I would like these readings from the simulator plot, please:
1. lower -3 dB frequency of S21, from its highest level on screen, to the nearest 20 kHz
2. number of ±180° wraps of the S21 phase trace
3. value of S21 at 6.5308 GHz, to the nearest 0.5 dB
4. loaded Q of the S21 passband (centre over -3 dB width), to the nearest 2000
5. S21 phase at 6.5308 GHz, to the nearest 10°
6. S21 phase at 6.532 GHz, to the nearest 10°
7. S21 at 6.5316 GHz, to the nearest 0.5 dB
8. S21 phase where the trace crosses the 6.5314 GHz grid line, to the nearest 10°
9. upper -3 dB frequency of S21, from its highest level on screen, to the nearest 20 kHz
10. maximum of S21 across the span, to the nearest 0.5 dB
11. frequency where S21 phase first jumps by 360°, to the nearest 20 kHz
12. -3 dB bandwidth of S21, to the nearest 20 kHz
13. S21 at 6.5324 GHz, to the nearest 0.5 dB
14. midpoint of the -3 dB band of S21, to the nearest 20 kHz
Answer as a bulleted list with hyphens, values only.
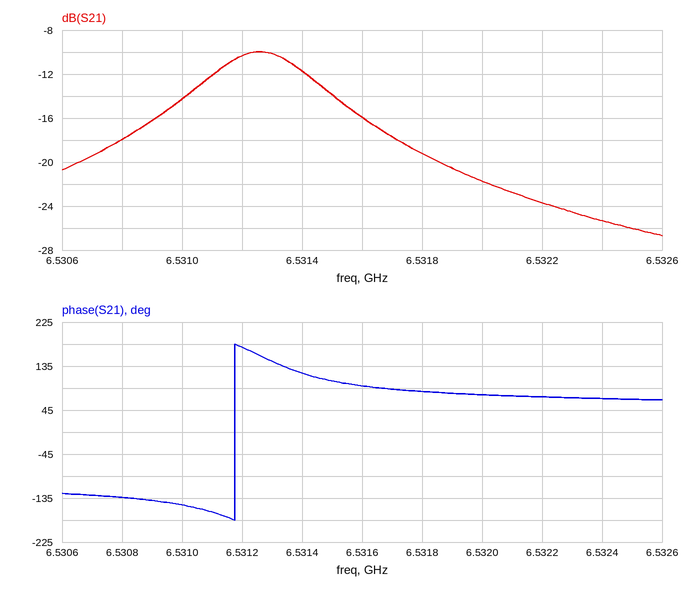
- 6.53106 GHz
- 1
- -18.0 dB
- 16000
- -130°
- 80°
- -16.0 dB
- 120°
- 6.53146 GHz
- -10.0 dB
- 6.53118 GHz
- 400 kHz
- -25.5 dB
- 6.53126 GHz
